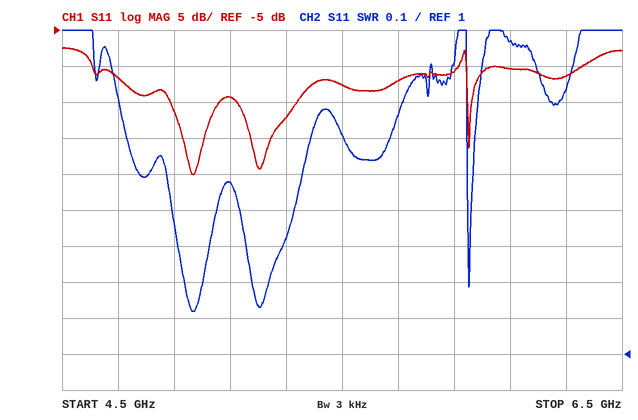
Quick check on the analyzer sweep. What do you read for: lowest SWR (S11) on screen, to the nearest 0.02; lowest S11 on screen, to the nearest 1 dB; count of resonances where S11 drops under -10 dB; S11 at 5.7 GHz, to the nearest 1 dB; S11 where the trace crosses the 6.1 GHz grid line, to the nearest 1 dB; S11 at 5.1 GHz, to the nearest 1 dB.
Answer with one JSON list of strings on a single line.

["1.12", "-25 dB", "3", "-12 dB", "-10 dB", "-14 dB"]
